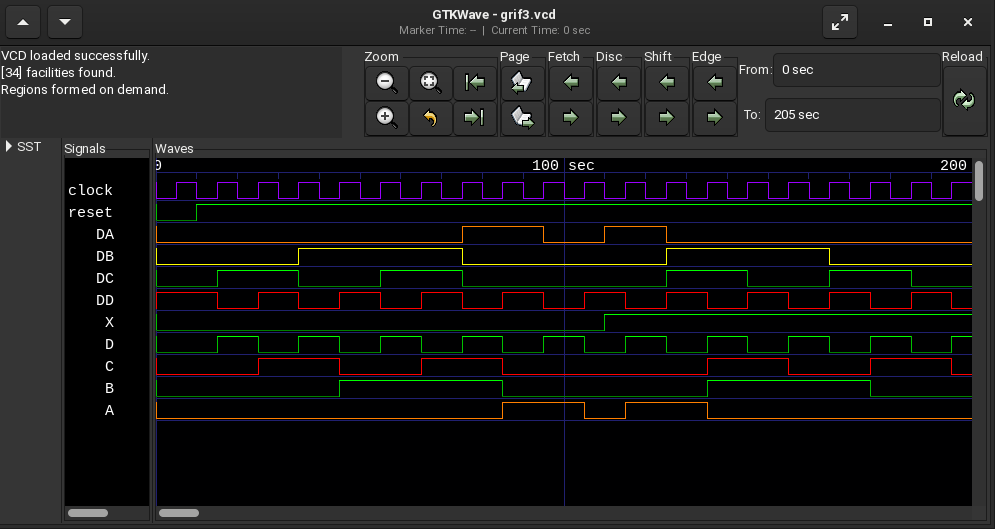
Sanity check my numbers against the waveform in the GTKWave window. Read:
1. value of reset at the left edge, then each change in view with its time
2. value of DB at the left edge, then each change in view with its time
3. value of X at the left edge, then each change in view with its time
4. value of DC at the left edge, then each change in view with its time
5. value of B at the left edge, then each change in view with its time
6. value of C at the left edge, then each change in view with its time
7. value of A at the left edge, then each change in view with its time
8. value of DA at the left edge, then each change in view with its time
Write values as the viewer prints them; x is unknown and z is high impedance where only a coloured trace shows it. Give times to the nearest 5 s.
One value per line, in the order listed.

0, 1 at 10 s
0, 1 at 35 s, 0 at 75 s, 1 at 125 s, 0 at 165 s
0, 1 at 110 s
0, 1 at 15 s, 0 at 35 s, 1 at 55 s, 0 at 75 s, 1 at 125 s, 0 at 145 s, 1 at 165 s, 0 at 185 s
0, 1 at 45 s, 0 at 85 s, 1 at 135 s, 0 at 175 s
0, 1 at 25 s, 0 at 45 s, 1 at 65 s, 0 at 85 s, 1 at 135 s, 0 at 155 s, 1 at 175 s, 0 at 195 s
0, 1 at 85 s, 0 at 105 s, 1 at 115 s, 0 at 135 s
0, 1 at 75 s, 0 at 95 s, 1 at 110 s, 0 at 125 s
